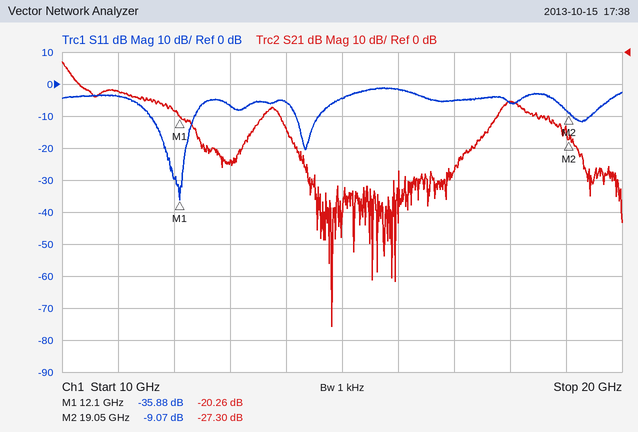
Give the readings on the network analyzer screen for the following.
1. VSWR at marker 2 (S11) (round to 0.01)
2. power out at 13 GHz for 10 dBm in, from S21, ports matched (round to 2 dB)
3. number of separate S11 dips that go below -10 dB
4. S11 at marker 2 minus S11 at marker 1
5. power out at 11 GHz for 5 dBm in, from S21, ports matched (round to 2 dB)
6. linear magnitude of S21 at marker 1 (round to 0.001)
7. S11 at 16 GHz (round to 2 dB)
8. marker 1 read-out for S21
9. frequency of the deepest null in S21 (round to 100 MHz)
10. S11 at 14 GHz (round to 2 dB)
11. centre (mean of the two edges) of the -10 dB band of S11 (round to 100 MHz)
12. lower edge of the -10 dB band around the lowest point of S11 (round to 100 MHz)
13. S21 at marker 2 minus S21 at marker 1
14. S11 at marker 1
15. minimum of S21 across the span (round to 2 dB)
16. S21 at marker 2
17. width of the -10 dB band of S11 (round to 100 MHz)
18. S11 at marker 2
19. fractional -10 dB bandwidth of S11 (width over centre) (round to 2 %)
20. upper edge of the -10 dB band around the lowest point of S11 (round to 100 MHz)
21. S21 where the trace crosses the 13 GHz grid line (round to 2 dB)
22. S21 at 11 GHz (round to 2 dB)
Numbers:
2.09
-24 dBm
3
26.81 dB
-8 dBm
0.097
-2 dB
-20.26 dB
14.8 GHz
-6 dB
12.0 GHz
11.6 GHz
-7.04 dB
-35.88 dB
-86 dB
-27.30 dB
800 MHz
-9.07 dB
6 %
12.4 GHz
-34 dB
-12 dB
